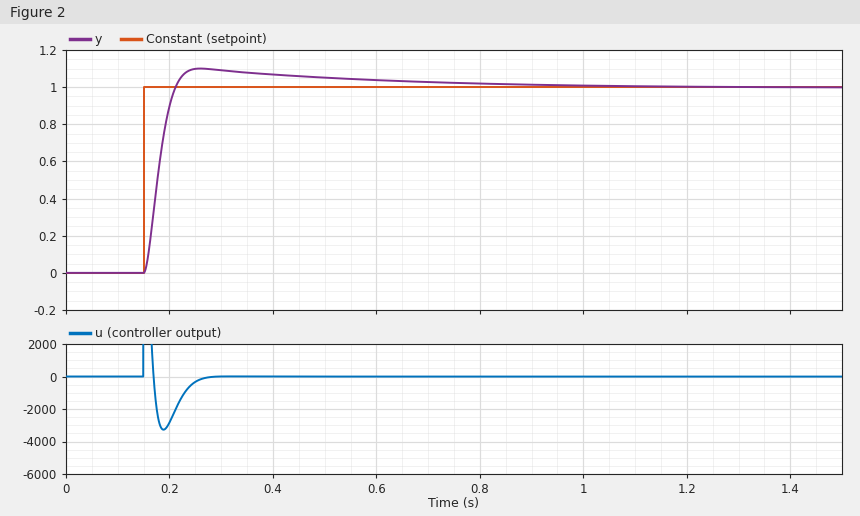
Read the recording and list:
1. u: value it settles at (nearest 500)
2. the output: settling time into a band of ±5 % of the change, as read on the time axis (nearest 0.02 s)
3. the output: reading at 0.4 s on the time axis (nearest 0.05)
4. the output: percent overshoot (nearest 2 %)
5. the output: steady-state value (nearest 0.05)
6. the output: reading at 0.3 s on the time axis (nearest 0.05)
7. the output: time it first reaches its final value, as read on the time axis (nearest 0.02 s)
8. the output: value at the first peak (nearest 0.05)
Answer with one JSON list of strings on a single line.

["0", "0.50 s", "1.05", "10 %", "1.00", "1.10", "0.22 s", "1.10"]
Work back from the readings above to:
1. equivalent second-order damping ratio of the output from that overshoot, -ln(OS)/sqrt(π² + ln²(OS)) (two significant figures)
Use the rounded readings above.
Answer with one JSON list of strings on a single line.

["0.59"]
